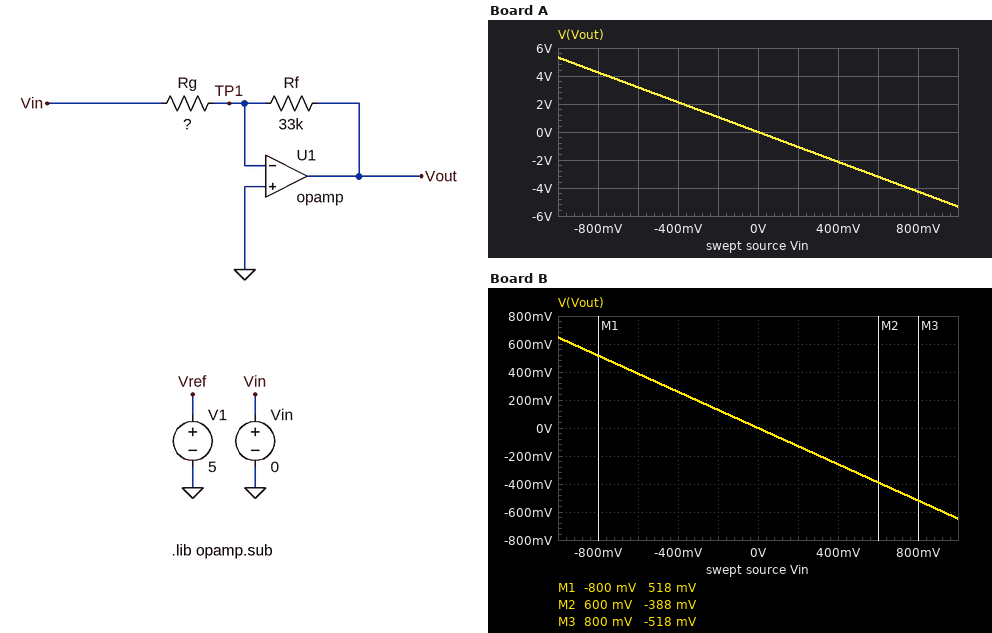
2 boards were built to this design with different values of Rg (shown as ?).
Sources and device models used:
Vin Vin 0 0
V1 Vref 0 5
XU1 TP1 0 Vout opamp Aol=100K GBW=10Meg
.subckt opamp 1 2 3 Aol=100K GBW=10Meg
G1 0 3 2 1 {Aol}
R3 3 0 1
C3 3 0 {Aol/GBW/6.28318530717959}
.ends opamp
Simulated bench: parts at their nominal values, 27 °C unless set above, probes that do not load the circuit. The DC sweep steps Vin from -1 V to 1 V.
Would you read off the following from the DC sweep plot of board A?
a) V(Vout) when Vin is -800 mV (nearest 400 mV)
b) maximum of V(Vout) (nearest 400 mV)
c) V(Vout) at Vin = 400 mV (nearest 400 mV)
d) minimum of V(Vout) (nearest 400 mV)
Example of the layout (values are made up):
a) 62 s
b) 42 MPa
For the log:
a) 4.4 V
b) 5.2 V
c) -2.0 V
d) -5.2 V
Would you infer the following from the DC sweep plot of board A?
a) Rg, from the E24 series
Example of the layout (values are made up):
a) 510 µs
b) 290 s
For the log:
a) 6.2 kΩ
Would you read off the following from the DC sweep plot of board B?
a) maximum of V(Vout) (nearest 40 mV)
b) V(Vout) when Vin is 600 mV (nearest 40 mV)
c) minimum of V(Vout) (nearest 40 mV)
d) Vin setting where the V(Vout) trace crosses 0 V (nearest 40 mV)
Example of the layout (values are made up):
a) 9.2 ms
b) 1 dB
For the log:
a) 640 mV
b) -400 mV
c) -640 mV
d) 0 V
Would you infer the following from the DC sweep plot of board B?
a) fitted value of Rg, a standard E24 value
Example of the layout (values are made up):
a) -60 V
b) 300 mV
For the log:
a) 51 kΩ
